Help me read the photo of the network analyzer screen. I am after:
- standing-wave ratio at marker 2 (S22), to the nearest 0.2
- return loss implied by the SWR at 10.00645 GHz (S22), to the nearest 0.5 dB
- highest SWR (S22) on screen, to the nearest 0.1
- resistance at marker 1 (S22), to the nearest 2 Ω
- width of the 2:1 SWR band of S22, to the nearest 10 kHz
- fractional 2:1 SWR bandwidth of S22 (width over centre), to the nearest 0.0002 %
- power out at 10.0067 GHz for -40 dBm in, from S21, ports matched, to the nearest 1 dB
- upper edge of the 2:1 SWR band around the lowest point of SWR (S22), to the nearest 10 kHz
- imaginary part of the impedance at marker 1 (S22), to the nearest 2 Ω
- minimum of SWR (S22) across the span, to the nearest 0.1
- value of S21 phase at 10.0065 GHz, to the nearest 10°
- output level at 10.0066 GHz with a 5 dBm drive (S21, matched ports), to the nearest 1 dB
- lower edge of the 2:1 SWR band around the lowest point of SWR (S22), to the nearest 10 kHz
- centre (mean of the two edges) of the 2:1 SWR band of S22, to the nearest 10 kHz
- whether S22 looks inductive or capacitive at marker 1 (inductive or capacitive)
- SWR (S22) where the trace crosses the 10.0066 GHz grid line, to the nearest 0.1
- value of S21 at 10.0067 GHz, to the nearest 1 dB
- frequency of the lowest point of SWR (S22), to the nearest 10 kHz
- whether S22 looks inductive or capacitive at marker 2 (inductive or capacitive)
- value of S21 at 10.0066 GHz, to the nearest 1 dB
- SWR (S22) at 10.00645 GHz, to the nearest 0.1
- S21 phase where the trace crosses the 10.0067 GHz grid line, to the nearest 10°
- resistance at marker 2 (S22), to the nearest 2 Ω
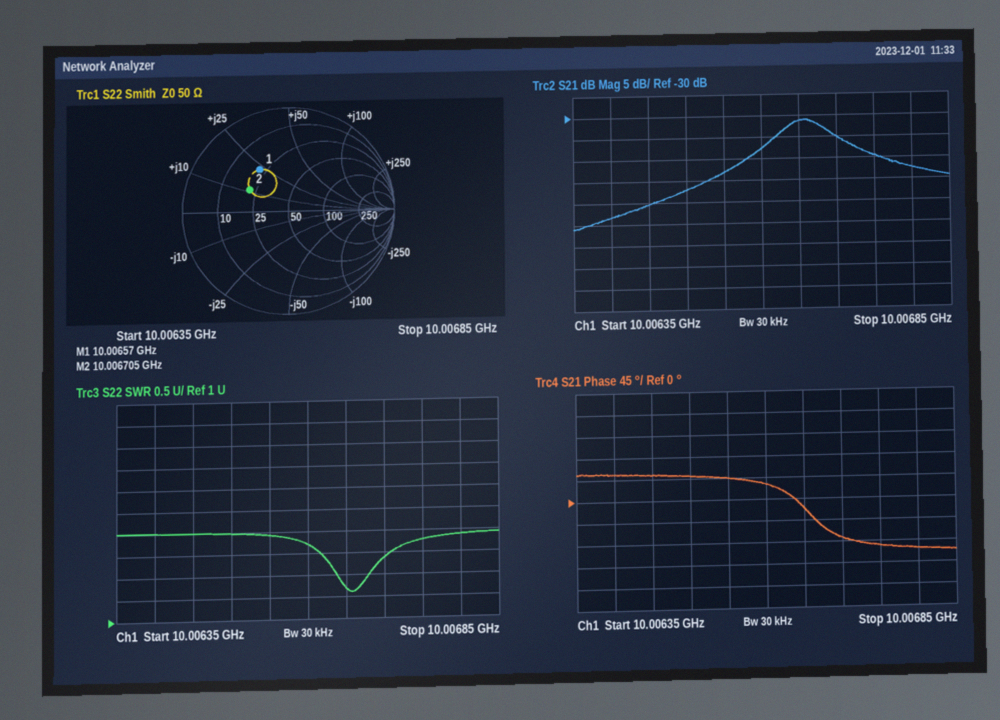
2.4
6.0 dB
3.0
22 Ω
40 kHz
0.0004 %
-75 dBm
10.00668 GHz
+22 Ω
1.6
50°
-33 dBm
10.00664 GHz
10.00666 GHz
inductive
2.7
-35 dB
10.00666 GHz
inductive
-38 dB
3.0
-80°
22 Ω
